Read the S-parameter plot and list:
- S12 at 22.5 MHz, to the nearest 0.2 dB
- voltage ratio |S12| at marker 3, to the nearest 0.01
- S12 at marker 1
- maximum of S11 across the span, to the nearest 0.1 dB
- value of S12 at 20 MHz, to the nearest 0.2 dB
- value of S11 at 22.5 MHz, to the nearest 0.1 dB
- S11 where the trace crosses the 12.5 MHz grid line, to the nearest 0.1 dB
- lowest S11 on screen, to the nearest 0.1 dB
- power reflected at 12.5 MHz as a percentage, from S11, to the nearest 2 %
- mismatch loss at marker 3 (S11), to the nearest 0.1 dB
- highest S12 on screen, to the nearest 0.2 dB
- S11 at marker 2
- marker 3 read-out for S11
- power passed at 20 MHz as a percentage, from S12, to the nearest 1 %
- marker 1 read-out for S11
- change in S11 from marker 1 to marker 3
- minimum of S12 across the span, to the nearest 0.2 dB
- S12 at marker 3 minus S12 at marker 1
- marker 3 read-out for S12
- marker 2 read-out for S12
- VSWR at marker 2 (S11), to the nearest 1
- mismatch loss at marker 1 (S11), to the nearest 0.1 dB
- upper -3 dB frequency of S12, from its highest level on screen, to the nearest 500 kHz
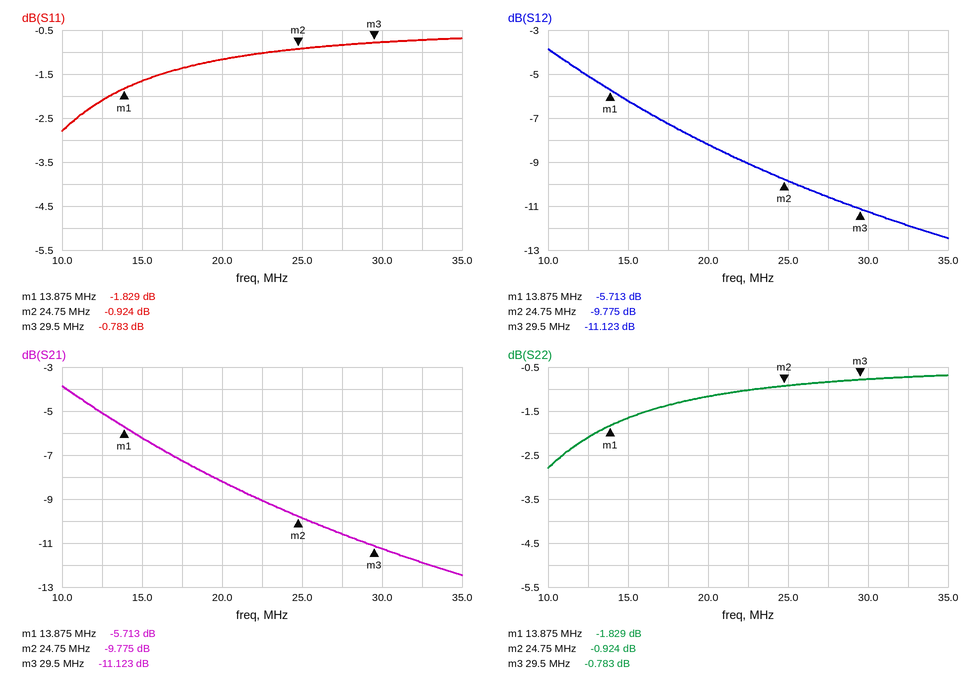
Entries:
-9.0 dB
0.28
-5.713 dB
-0.7 dB
-8.2 dB
-1.0 dB
-2.1 dB
-2.8 dB
62 %
7.8 dB
-3.8 dB
-0.924 dB
-0.783 dB
15 %
-1.829 dB
1.046 dB
-12.4 dB
-5.410 dB
-11.123 dB
-9.775 dB
19
4.6 dB
16.5 MHz
